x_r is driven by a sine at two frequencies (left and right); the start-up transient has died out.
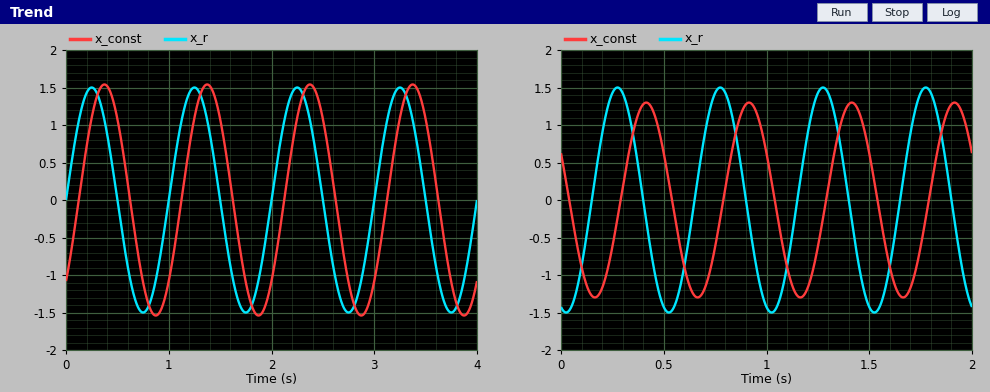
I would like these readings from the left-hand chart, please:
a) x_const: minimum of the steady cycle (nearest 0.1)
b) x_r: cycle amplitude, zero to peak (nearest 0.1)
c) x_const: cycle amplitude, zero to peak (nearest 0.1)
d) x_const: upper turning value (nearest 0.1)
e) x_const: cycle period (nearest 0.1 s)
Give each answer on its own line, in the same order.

-1.5
1.5
1.5
1.5
1.0 s
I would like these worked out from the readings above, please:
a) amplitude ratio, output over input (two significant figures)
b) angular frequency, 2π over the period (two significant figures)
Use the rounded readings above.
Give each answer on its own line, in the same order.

1.0
6.3 rad/s
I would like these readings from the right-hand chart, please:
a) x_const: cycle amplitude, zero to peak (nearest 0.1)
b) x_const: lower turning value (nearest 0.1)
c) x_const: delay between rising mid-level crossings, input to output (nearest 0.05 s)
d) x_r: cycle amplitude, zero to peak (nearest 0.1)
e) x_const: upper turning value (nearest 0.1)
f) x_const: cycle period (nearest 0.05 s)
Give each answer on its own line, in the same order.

1.3
-1.3
0.15 s
1.5
1.3
0.50 s
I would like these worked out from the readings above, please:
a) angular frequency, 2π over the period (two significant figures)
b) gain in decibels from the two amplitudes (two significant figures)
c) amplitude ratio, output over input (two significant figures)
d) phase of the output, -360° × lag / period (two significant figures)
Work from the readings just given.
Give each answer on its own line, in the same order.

13 rad/s
-1.2 dB
0.87
-110°
